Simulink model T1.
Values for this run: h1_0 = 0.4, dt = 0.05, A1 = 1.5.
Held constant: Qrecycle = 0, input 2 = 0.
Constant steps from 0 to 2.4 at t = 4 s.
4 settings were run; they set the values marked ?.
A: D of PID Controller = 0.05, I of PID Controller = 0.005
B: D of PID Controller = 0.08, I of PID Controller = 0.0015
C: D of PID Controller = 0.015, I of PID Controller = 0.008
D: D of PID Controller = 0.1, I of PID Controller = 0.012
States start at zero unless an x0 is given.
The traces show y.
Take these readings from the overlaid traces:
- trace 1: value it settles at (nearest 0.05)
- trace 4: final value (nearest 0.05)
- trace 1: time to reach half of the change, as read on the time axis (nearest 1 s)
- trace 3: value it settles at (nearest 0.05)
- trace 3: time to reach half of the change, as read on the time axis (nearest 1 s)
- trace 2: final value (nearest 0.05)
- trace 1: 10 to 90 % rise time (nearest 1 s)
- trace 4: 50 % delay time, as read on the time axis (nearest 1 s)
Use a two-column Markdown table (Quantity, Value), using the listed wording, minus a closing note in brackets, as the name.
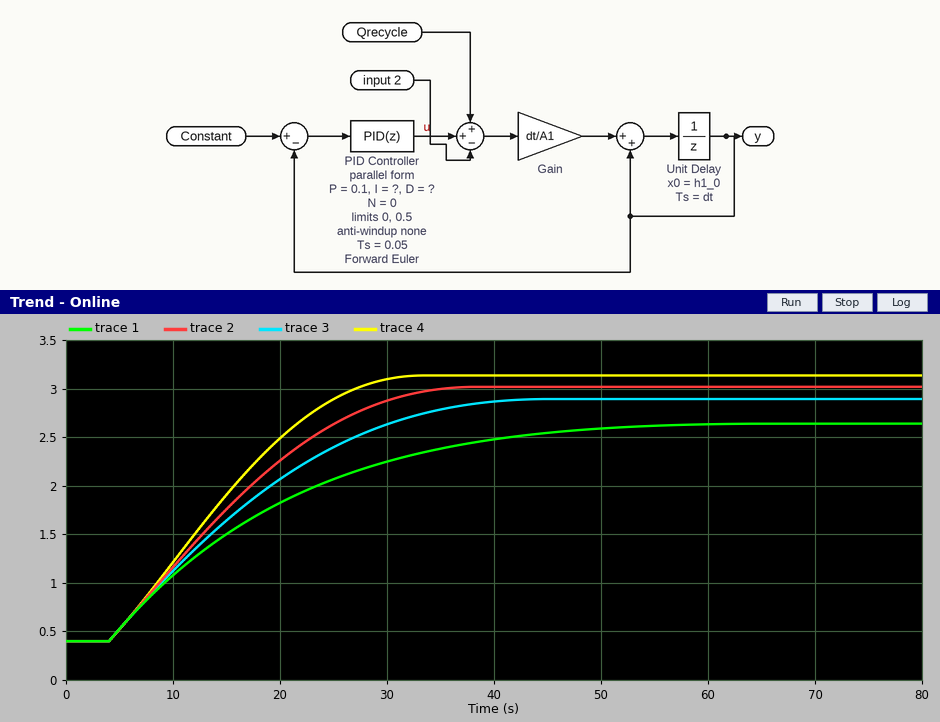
| Quantity | Value |
|---|---|
| trace 1: value it settles at | 2.65 |
| trace 4: final value | 3.15 |
| trace 1: time to reach half of the change, as read on the time axis | 15 s |
| trace 3: value it settles at | 2.90 |
| trace 3: time to reach half of the change, as read on the time axis | 15 s |
| trace 2: final value | 3.00 |
| trace 1: 10 to 90 % rise time | 31 s |
| trace 4: 50 % delay time, as read on the time axis | 14 s |
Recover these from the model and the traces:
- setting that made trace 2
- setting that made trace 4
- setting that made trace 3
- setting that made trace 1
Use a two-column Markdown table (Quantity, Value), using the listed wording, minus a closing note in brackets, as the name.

| Quantity | Value |
|---|---|
| setting that made trace 2 | C |
| setting that made trace 4 | D |
| setting that made trace 3 | A |
| setting that made trace 1 | B |
